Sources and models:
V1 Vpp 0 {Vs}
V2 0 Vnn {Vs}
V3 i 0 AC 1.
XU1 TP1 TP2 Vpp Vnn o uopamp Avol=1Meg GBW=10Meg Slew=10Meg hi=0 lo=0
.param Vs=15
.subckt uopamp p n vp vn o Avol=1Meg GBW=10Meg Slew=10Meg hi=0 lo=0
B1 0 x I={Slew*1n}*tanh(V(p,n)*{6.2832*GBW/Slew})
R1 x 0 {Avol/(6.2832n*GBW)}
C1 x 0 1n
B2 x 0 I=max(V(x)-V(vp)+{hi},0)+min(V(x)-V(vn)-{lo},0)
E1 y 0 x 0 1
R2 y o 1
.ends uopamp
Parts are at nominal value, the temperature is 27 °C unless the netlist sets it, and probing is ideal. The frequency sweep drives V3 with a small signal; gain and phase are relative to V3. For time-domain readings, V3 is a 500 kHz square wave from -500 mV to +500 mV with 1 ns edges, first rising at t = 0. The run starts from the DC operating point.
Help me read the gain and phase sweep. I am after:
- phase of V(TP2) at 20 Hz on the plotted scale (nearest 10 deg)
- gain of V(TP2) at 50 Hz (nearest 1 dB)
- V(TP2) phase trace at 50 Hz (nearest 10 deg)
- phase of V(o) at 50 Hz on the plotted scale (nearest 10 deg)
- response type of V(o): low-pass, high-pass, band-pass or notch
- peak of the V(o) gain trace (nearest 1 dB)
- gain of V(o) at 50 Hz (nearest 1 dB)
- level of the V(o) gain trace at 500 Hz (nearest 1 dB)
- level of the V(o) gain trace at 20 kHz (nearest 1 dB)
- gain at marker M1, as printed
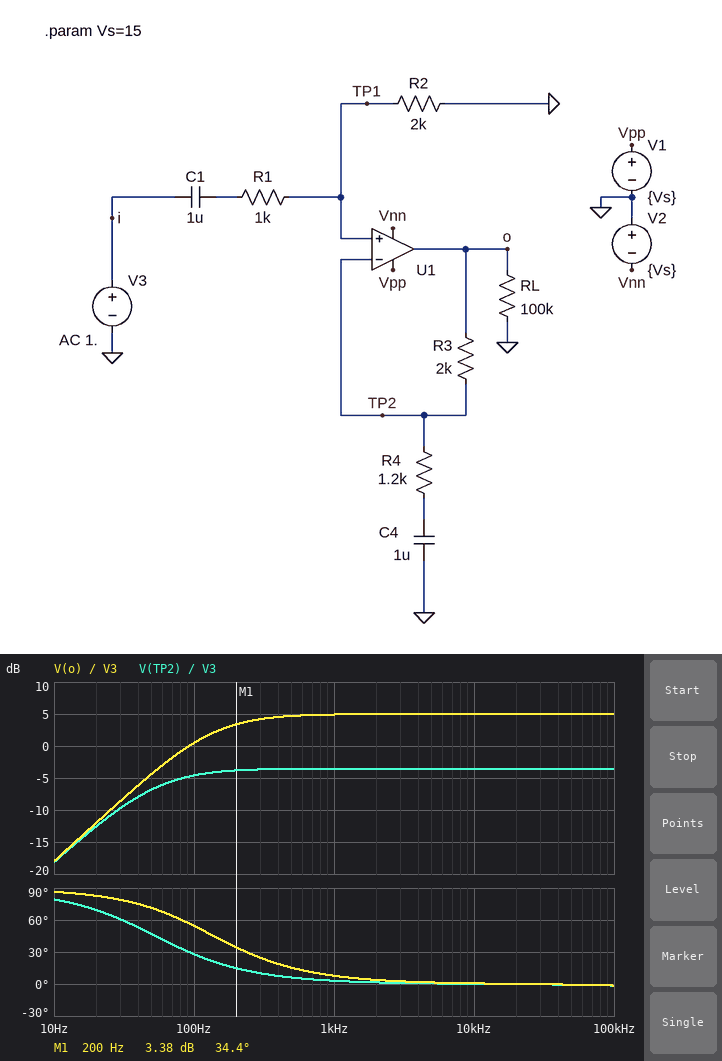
70 deg
-7 dB
50 deg
70 deg
high-pass
5 dB
-4 dB
5 dB
5 dB
3.38 dB
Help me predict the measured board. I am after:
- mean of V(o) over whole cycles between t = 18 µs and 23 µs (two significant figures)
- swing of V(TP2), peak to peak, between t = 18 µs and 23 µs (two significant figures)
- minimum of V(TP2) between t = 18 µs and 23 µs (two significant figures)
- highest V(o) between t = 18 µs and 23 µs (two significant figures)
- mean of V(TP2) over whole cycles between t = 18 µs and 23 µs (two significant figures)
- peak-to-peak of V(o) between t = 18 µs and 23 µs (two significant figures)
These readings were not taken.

870 mV
670 mV
-2.4 mV
1.8 V
330 mV
1.8 V
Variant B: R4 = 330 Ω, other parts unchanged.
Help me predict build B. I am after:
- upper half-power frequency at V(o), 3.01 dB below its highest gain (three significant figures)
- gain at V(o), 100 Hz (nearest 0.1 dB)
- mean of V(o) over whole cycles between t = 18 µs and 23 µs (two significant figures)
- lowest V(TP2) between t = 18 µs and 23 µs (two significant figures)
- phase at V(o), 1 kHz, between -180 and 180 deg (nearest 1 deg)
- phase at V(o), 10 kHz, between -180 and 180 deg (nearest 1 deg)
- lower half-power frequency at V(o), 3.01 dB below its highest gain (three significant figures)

1.42 MHz
0.2 dB
2.2 V
-1.7 mV
25 deg
2 deg
478 Hz
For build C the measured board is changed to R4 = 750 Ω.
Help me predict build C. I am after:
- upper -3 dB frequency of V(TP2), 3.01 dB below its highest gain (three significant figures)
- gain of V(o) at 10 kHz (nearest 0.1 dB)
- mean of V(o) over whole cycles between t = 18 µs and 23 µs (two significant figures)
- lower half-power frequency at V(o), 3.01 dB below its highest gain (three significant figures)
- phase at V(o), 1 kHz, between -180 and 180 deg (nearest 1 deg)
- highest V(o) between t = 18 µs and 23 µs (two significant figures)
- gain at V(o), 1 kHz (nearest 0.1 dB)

2.73 MHz
7.8 dB
1.2 V
210 Hz
12 deg
2.4 V
7.6 dB
